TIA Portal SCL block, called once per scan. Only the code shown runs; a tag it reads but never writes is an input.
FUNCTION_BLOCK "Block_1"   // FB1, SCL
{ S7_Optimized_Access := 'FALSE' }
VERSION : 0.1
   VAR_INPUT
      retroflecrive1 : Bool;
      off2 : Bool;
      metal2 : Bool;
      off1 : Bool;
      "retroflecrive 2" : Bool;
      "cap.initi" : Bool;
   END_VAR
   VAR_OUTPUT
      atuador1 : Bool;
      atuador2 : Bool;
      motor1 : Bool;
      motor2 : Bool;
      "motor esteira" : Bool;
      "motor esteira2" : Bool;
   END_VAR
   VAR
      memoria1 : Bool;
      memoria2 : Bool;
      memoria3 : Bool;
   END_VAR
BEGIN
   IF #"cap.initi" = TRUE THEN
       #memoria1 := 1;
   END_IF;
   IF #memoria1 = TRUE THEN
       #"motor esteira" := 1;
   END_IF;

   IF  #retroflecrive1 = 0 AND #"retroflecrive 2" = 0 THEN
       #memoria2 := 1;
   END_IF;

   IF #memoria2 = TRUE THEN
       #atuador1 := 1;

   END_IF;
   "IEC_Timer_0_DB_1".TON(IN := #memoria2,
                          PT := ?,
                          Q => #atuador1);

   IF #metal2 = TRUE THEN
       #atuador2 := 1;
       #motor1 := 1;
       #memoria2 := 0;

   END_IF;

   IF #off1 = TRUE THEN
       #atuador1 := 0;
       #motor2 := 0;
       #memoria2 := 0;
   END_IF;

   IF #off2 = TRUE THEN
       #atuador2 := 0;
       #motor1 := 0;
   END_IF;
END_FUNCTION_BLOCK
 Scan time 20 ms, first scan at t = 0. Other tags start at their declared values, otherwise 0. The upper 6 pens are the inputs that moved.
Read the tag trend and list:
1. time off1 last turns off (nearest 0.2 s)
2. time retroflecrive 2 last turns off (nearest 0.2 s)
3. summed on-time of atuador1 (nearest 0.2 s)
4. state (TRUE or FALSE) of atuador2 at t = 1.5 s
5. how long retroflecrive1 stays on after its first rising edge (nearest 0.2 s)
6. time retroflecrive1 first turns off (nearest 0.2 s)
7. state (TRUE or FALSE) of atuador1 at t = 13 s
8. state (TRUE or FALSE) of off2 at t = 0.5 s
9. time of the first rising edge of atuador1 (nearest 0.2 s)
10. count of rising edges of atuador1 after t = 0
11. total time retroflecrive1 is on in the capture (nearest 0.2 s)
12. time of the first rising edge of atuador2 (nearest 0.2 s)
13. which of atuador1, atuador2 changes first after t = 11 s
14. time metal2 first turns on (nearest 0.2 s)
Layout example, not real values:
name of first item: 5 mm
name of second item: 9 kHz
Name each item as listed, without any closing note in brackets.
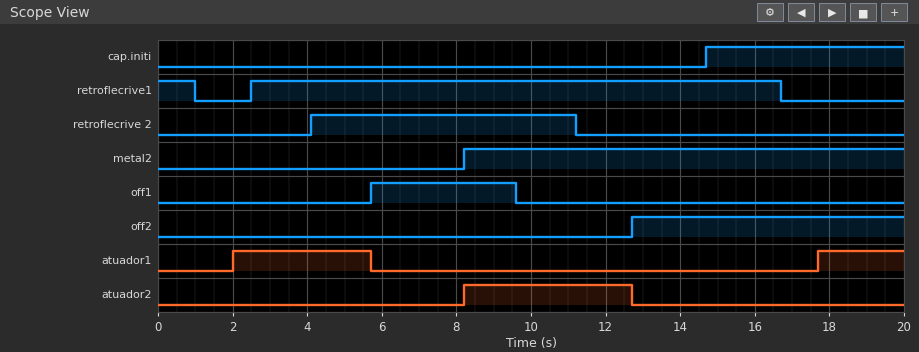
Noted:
time off1 last turns off: 9.6 s
time retroflecrive 2 last turns off: 11.2 s
summed on-time of atuador1: 6.0 s
state (TRUE or FALSE) of atuador2 at t = 1.5 s: FALSE
how long retroflecrive1 stays on after its first rising edge: 14.2 s
time retroflecrive1 first turns off: 1.0 s
state (TRUE or FALSE) of atuador1 at t = 13 s: FALSE
state (TRUE or FALSE) of off2 at t = 0.5 s: FALSE
time of the first rising edge of atuador1: 2.0 s
count of rising edges of atuador1 after t = 0: 2
total time retroflecrive1 is on in the capture: 15.2 s
time of the first rising edge of atuador2: 8.2 s
which of atuador1, atuador2 changes first after t = 11 s: atuador2
time metal2 first turns on: 8.2 s
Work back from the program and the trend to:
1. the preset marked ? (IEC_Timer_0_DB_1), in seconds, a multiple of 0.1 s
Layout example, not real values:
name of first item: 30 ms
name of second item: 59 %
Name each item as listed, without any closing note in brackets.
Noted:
the preset marked ? (IEC_Timer_0_DB_1), in seconds, a multiple of 0.1 s: 1.0 s
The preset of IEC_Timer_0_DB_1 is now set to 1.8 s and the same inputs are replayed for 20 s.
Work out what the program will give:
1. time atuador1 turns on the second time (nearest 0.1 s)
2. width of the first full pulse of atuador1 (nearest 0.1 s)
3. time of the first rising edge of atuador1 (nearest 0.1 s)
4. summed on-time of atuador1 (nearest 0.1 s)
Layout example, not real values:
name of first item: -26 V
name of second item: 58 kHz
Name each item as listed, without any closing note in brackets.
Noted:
time atuador1 turns on the second time: 18.5 s
width of the first full pulse of atuador1: 2.9 s
time of the first rising edge of atuador1: 2.8 s
summed on-time of atuador1: 4.4 s
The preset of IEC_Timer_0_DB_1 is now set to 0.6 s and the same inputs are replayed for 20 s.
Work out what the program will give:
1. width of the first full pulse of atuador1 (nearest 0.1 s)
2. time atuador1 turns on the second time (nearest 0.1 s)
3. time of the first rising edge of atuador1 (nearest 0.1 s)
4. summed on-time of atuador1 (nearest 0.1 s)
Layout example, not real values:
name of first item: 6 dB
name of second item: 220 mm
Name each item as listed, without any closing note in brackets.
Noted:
width of the first full pulse of atuador1: 4.1 s
time atuador1 turns on the second time: 17.3 s
time of the first rising edge of atuador1: 1.6 s
summed on-time of atuador1: 6.8 s
